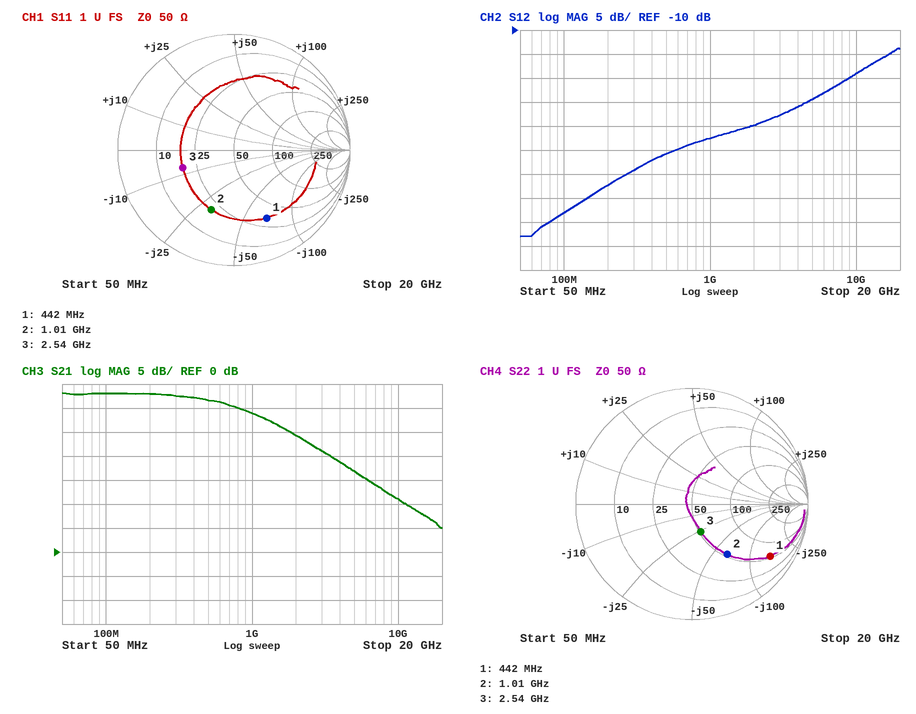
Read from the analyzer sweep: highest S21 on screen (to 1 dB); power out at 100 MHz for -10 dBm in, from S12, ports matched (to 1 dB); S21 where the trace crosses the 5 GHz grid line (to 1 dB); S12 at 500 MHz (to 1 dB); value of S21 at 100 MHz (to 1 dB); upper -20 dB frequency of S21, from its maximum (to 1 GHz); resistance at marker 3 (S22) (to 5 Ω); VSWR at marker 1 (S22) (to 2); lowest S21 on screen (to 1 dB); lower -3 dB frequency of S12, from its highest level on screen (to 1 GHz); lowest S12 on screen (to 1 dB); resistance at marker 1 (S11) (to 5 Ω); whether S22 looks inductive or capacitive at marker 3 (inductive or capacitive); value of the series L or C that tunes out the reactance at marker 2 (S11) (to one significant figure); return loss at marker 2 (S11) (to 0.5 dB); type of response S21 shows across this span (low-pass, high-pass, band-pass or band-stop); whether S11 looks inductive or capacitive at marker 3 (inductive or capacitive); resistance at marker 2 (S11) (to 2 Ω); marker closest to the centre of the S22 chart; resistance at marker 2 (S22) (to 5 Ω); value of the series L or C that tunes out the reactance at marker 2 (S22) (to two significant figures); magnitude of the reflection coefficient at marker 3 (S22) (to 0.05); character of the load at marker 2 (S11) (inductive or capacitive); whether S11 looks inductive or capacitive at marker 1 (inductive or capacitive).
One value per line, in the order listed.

33 dB
-58 dBm
17 dB
-36 dB
33 dB
8 GHz
50 Ω
10
5 dB
13 GHz
-53 dB
35 Ω
capacitive
5 nH
5.0 dB
low-pass
capacitive
20 Ω
marker 3
55 Ω
10 nH
0.25
capacitive
capacitive
